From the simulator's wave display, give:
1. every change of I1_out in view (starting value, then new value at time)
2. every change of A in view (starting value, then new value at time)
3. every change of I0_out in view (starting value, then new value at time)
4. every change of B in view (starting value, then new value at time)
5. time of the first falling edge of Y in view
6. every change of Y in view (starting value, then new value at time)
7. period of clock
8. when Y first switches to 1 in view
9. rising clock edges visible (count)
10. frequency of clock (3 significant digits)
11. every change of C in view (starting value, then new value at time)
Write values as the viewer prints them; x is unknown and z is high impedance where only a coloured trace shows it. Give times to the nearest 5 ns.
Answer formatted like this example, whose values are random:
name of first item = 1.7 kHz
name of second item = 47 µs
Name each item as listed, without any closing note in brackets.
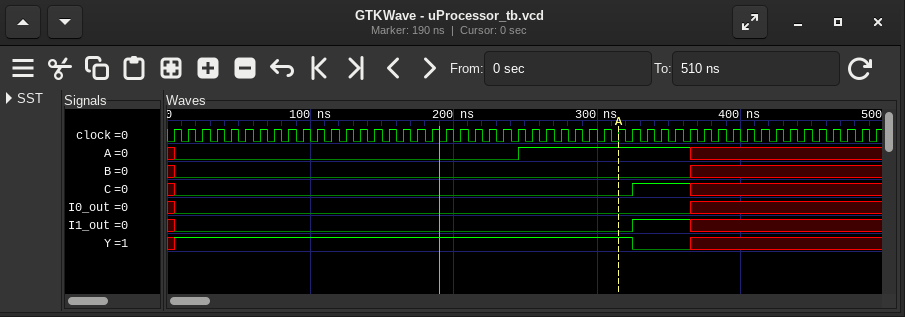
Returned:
every change of I1_out in view = x, 0 at 5 ns, 1 at 325 ns, x at 365 ns
every change of A in view = x, 0 at 5 ns, 1 at 245 ns, x at 365 ns
every change of I0_out in view = x, 0 at 5 ns, x at 365 ns
every change of B in view = x, 0 at 5 ns, x at 365 ns
time of the first falling edge of Y in view = 325 ns
every change of Y in view = x, 1 at 5 ns, 0 at 325 ns, x at 365 ns
period of clock = 10 ns
when Y first switches to 1 in view = 5 ns
rising clock edges visible = 50
frequency of clock = 100 MHz
every change of C in view = x, 0 at 5 ns, 1 at 325 ns, x at 365 ns
